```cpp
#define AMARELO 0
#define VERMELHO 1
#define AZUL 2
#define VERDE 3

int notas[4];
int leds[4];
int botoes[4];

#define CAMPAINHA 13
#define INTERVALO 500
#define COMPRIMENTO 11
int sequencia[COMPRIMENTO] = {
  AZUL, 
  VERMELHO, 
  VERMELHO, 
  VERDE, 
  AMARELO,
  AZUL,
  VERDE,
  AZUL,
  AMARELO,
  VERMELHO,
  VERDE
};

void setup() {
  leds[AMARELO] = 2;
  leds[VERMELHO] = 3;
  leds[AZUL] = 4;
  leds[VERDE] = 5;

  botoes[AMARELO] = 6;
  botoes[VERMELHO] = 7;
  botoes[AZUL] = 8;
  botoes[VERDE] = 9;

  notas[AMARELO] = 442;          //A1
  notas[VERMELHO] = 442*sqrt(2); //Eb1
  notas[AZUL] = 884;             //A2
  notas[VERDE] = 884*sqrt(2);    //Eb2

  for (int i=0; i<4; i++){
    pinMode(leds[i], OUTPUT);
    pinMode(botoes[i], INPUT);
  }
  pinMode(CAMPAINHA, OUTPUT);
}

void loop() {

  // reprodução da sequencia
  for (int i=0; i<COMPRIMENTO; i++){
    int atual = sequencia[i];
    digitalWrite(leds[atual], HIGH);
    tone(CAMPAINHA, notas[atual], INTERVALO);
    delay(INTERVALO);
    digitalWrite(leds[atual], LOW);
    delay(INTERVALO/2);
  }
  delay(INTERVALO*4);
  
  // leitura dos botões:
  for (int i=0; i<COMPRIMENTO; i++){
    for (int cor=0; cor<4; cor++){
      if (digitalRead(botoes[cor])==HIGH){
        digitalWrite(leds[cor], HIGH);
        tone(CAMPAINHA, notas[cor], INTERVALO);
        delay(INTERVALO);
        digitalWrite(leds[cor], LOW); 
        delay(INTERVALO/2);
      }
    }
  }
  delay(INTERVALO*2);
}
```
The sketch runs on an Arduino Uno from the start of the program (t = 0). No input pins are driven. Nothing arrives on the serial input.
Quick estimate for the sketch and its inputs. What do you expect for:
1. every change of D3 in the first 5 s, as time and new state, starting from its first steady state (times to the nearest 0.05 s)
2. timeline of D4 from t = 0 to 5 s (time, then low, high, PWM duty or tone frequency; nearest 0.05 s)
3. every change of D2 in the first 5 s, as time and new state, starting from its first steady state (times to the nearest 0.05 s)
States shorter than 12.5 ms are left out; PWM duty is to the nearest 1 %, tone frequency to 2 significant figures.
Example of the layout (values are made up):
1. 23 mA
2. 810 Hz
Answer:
1. 0 s low; 0.75 s high; 1.25 s low; 1.5 s high; 2 s low
2. 0 s high; 0.5 s low; 3.75 s high; 4.25 s low
3. 0 s low; 3 s high; 3.5 s low
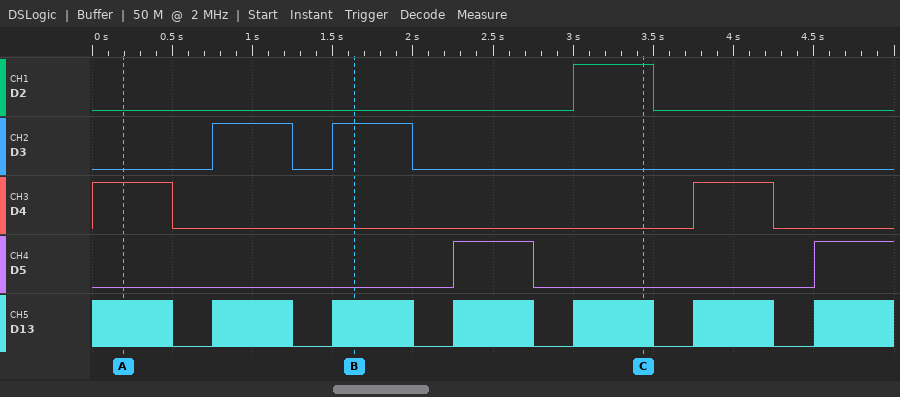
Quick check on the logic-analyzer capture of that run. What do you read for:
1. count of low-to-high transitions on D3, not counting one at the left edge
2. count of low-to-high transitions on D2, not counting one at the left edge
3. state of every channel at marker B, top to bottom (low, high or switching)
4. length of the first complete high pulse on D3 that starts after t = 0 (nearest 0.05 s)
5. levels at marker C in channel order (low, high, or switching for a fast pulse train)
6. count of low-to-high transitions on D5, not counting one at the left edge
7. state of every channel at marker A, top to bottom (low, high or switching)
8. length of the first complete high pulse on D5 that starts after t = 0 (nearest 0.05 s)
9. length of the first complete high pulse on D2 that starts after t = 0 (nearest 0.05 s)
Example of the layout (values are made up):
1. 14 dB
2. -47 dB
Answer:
1. 2
2. 1
3. D2 low, D3 high, D4 low, D5 low, D13 switching
4. 0.50 s
5. D2 high, D3 low, D4 low, D5 low, D13 switching
6. 2
7. D2 low, D3 low, D4 high, D5 low, D13 switching
8. 0.50 s
9. 0.50 s
